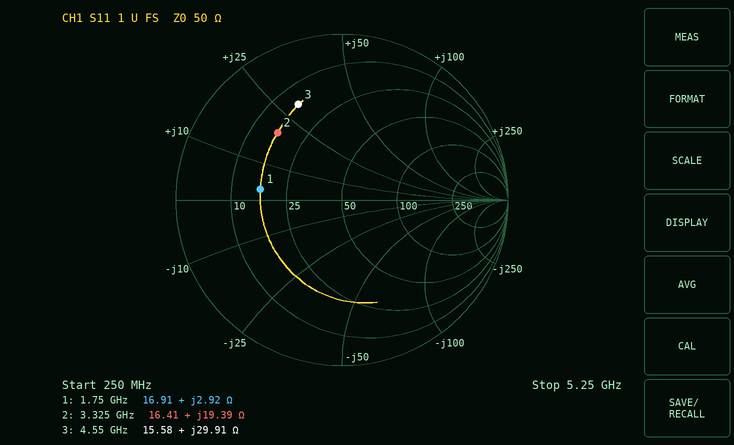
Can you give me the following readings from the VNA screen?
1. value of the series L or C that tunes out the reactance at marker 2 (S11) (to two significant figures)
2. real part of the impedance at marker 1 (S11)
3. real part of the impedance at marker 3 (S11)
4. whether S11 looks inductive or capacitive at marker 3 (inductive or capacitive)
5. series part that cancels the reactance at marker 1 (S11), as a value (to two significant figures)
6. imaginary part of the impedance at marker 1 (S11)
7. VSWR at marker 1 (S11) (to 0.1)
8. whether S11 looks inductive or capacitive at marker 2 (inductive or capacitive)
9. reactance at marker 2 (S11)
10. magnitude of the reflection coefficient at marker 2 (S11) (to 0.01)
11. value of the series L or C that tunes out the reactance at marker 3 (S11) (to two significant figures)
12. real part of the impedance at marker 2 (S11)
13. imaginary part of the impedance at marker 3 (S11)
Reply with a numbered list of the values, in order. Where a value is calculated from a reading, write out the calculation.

1. C = 1/(2π × 3.325 GHz × 19.39 Ω) ≈ 2.5 pF
2. 16.91 Ω
3. 15.58 Ω
4. inductive
5. C = 1/(2π × 1.75 GHz × 2.92 Ω) ≈ 31 pF
6. +2.92 Ω
7. 3.0
8. inductive
9. +19.39 Ω
10. 0.56
11. C = 1/(2π × 4.55 GHz × 29.91 Ω) ≈ 1.2 pF
12. 16.41 Ω
13. +29.91 Ω
